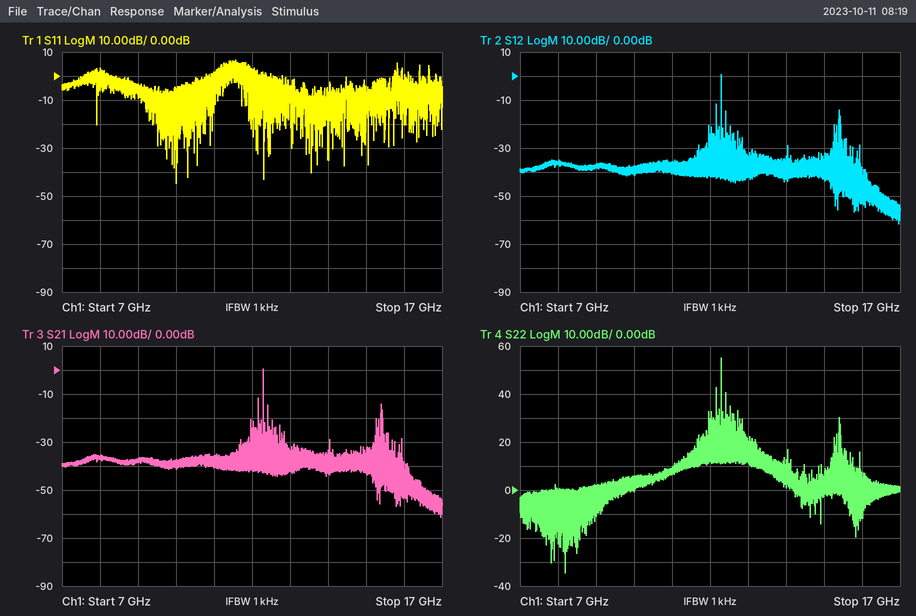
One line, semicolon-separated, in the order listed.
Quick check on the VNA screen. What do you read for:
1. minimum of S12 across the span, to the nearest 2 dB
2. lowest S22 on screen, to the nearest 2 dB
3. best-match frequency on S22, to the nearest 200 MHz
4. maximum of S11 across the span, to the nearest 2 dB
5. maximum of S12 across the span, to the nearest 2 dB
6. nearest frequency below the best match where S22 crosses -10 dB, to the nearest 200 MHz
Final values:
-62 dB; -34 dB; 8.2 GHz; 6 dB; 0 dB; 8.2 GHz
